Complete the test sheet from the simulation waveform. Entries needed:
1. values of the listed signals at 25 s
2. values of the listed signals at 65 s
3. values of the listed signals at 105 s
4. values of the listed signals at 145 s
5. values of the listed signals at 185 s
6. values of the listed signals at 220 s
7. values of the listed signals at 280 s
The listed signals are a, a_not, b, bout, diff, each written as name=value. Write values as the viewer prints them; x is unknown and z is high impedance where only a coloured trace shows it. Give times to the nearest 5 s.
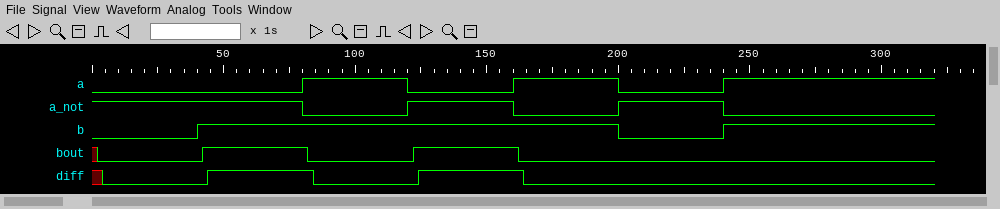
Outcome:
a=0, a_not=1, b=0, bout=0, diff=0
a=0, a_not=1, b=1, bout=1, diff=1
a=1, a_not=0, b=1, bout=0, diff=0
a=0, a_not=1, b=1, bout=1, diff=1
a=1, a_not=0, b=1, bout=0, diff=0
a=0, a_not=1, b=0, bout=0, diff=0
a=1, a_not=0, b=1, bout=0, diff=0
